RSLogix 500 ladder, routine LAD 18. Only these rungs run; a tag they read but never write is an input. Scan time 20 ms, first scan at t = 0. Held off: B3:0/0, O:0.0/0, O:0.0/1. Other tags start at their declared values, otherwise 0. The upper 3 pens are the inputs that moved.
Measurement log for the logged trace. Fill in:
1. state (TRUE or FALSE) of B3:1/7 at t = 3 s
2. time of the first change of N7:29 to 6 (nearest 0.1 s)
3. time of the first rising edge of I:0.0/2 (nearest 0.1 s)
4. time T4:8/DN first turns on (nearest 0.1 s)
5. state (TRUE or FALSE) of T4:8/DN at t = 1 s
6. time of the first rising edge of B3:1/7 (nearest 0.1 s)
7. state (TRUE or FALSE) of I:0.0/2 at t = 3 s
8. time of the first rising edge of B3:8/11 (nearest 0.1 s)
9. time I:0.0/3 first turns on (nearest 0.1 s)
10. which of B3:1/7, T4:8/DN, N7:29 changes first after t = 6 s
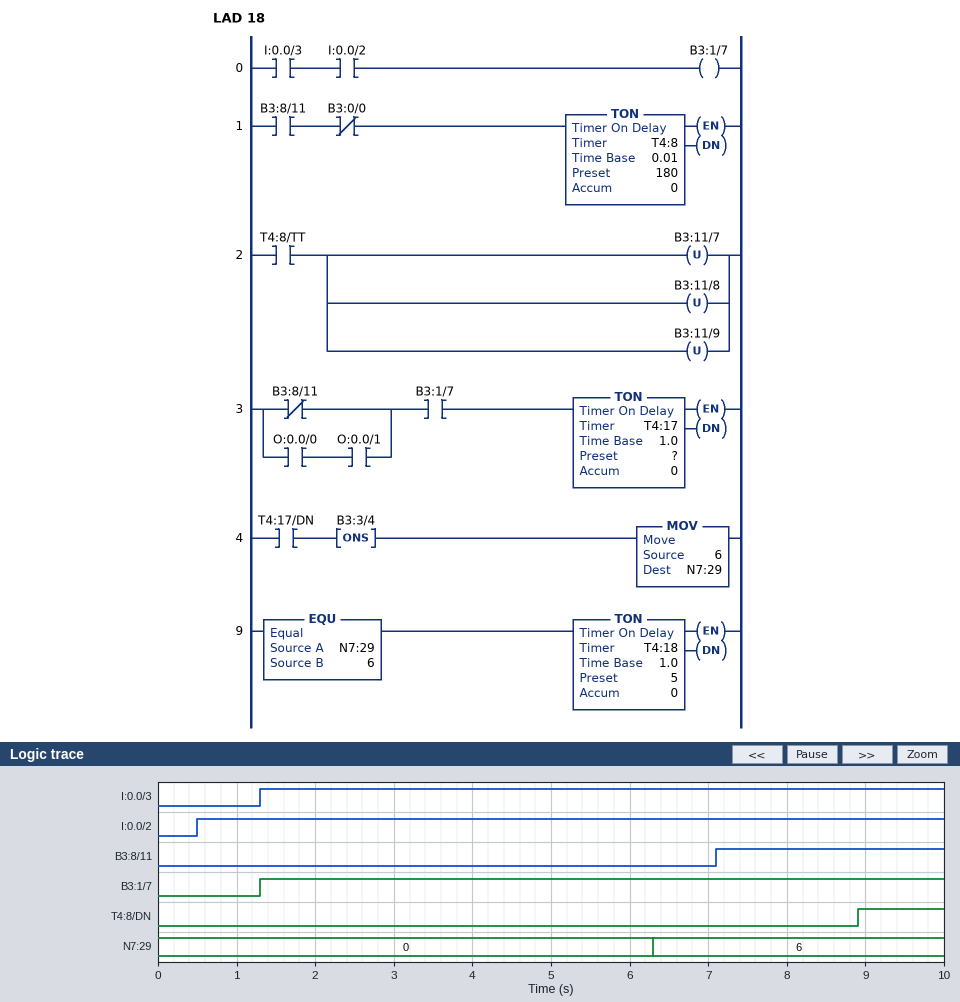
TRUE
6.3 s
0.5 s
8.9 s
FALSE
1.3 s
TRUE
7.1 s
1.3 s
N7:29
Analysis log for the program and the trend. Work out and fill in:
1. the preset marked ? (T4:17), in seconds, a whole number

5 s
